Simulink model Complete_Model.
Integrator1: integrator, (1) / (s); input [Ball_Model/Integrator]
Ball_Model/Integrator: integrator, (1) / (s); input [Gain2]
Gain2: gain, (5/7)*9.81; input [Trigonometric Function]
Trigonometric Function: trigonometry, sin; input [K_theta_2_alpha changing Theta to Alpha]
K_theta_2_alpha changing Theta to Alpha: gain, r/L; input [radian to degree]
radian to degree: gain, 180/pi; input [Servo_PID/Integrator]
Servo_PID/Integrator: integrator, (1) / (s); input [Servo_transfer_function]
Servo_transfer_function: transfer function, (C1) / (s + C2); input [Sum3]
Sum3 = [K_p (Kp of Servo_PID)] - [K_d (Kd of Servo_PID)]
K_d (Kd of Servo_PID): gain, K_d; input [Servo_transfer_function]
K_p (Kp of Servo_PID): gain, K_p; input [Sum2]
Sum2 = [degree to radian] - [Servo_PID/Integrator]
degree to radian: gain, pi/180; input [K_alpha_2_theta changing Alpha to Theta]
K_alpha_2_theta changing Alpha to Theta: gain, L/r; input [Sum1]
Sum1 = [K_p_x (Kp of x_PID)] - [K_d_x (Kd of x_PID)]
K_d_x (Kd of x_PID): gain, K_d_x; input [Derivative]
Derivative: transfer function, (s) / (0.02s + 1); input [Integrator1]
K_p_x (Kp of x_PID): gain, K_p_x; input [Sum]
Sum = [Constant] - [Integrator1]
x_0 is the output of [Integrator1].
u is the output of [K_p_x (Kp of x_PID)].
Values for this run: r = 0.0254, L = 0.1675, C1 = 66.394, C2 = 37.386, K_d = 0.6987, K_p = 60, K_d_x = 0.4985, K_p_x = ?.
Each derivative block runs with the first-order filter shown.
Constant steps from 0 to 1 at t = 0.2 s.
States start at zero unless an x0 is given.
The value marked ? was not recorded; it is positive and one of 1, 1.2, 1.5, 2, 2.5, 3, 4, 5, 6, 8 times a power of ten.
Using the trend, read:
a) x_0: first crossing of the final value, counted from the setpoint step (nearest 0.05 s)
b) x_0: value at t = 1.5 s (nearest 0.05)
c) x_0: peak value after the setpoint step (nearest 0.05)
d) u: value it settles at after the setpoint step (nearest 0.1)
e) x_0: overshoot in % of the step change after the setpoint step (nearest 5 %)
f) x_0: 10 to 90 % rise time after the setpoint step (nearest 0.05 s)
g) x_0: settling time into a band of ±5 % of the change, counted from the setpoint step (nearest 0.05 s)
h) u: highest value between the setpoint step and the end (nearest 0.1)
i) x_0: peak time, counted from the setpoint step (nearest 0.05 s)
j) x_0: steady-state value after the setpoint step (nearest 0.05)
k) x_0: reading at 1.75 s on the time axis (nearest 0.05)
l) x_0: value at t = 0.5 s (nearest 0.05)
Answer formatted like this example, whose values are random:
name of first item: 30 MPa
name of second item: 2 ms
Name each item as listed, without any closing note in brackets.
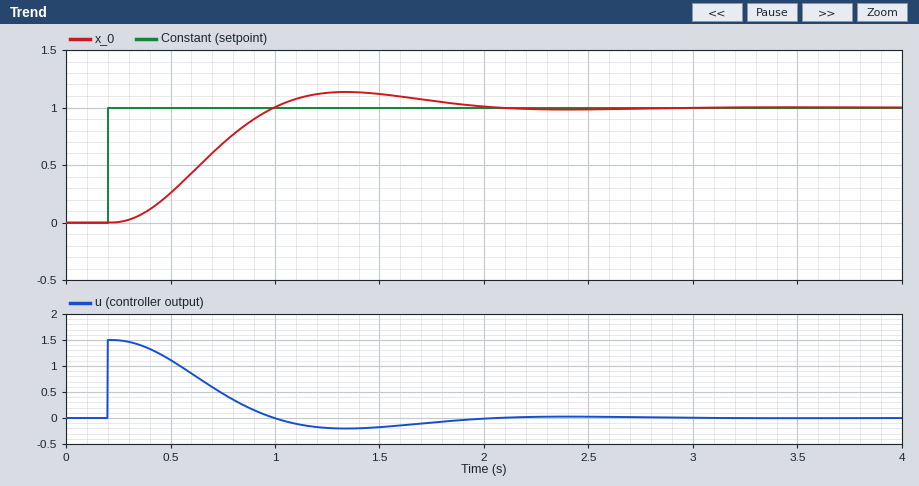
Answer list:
x_0: first crossing of the final value, counted from the setpoint step: 0.80 s
x_0: value at t = 1.5 s: 1.10
x_0: peak value after the setpoint step: 1.15
u: value it settles at after the setpoint step: 0.0
x_0: overshoot in % of the step change after the setpoint step: 15 %
x_0: 10 to 90 % rise time after the setpoint step: 0.50 s
x_0: settling time into a band of ±5 % of the change, counted from the setpoint step: 1.60 s
u: highest value between the setpoint step and the end: 1.5
x_0: peak time, counted from the setpoint step: 1.15 s
x_0: steady-state value after the setpoint step: 1.00
x_0: reading at 1.75 s on the time axis: 1.05
x_0: value at t = 0.5 s: 0.25
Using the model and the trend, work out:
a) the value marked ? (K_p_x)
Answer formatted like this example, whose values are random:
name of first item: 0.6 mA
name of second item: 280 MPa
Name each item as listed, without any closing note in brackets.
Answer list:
the value marked ?: 1.5
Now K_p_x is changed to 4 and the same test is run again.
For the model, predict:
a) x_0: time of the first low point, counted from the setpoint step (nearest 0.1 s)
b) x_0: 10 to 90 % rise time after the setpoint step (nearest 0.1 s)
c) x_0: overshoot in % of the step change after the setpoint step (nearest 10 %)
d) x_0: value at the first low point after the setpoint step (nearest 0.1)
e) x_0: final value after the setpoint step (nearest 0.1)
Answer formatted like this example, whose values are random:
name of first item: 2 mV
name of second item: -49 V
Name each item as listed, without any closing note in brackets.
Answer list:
x_0: time of the first low point, counted from the setpoint step: 0.8 s
x_0: 10 to 90 % rise time after the setpoint step: 0.3 s
x_0: overshoot in % of the step change after the setpoint step: 40 %
x_0: value at the first low point after the setpoint step: -0.8
x_0: final value after the setpoint step: -0.6
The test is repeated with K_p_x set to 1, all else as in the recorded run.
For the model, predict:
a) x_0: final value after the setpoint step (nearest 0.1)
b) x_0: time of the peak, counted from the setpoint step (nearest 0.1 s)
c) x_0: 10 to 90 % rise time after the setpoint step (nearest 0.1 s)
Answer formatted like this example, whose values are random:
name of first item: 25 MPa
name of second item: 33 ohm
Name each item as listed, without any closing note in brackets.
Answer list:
x_0: final value after the setpoint step: 1.0
x_0: time of the peak, counted from the setpoint step: 1.5 s
x_0: 10 to 90 % rise time after the setpoint step: 0.7 s
